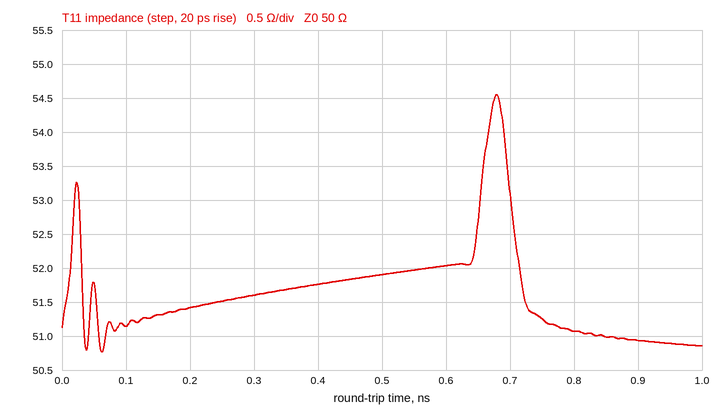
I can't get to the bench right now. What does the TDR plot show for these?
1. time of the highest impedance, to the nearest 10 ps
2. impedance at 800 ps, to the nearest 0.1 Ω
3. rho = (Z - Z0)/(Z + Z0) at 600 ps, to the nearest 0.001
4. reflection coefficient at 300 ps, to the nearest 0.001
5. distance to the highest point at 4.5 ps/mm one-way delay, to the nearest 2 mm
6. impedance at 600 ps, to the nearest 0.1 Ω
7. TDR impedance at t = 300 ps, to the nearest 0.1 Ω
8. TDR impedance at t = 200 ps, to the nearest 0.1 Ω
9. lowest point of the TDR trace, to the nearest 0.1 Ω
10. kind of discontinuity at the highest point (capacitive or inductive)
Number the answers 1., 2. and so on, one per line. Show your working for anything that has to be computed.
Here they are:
1. 680 ps
2. 51.1 Ω
3. (52 − 50)/(52 + 50) ≈ +0.020
4. (51.6 − 50)/(51.6 + 50) ≈ +0.016
5. 680 ps / 2 / 4.5 ps/mm ≈ 76 mm
6. 52.0 Ω
7. 51.6 Ω
8. 51.4 Ω
9. 50.8 Ω
10. inductive
